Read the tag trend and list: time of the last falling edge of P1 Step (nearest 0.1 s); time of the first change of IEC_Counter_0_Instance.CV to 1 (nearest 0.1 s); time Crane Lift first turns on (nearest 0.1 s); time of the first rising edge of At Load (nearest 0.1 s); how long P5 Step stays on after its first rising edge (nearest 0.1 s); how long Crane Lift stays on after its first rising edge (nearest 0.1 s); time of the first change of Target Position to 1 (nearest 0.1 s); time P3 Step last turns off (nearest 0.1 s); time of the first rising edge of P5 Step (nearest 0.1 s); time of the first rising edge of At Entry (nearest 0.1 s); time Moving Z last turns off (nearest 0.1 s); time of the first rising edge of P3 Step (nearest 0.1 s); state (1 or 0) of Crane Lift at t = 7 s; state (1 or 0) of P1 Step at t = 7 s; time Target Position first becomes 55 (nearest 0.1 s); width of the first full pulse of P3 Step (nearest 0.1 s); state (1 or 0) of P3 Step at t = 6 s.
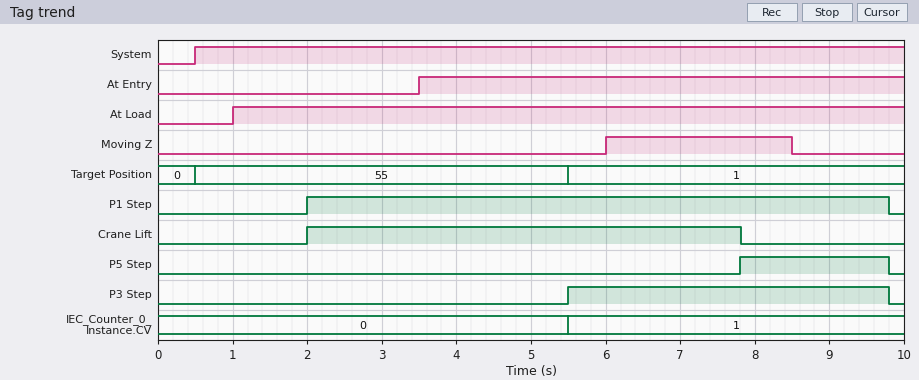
9.8 s
5.5 s
2.0 s
1.0 s
2.0 s
5.8 s
5.5 s
9.8 s
7.8 s
3.5 s
8.5 s
5.5 s
1
1
0.5 s
4.3 s
1
